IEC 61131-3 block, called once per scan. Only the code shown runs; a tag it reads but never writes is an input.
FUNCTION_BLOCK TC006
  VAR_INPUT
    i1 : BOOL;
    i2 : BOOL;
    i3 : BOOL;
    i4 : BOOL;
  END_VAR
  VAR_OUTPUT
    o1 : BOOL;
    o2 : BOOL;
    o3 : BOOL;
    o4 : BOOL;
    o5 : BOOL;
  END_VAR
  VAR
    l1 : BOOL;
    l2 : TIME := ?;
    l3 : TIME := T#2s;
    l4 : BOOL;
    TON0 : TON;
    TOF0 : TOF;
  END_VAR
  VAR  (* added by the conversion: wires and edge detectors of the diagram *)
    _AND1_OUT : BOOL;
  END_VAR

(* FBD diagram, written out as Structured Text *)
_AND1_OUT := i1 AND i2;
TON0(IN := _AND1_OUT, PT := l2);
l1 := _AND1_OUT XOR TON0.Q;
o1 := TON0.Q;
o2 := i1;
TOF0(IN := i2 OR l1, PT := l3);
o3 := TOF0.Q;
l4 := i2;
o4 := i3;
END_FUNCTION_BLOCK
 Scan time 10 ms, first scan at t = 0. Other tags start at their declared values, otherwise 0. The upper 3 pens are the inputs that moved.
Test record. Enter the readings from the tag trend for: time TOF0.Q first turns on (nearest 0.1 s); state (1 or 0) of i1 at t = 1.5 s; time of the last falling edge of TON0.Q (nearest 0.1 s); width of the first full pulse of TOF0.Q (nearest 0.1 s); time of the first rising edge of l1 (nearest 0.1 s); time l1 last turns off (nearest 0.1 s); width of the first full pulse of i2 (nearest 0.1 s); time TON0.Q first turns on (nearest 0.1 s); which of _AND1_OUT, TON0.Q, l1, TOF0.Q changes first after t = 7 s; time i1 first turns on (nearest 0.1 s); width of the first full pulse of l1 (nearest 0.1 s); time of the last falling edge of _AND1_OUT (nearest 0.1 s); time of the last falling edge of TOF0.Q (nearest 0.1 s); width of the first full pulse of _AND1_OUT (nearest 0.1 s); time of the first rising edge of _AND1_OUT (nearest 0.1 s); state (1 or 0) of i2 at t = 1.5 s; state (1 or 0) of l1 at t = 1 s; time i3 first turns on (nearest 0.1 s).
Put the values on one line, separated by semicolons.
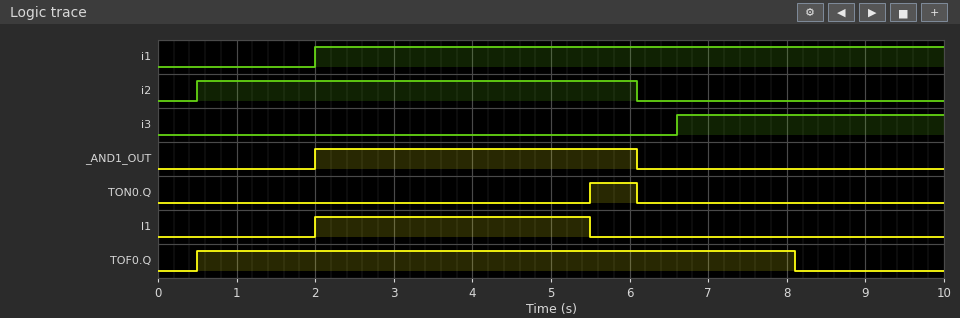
0.5 s; 0; 6.1 s; 7.6 s; 2.0 s; 5.5 s; 5.6 s; 5.5 s; TOF0.Q; 2.0 s; 3.5 s; 6.1 s; 8.1 s; 4.1 s; 2.0 s; 1; 0; 6.6 s
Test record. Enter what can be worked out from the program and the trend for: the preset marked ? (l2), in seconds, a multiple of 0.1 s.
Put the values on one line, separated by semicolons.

3.5 s
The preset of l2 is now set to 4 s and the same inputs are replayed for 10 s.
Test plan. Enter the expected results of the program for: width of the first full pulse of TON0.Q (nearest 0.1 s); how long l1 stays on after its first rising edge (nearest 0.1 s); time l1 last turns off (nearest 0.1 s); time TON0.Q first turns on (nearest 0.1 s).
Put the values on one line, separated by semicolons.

0.1 s; 4.0 s; 6.0 s; 6.0 s
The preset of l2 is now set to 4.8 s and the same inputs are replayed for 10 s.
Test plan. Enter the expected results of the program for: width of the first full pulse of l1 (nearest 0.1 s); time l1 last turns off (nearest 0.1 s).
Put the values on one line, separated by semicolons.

4.1 s; 6.1 s
